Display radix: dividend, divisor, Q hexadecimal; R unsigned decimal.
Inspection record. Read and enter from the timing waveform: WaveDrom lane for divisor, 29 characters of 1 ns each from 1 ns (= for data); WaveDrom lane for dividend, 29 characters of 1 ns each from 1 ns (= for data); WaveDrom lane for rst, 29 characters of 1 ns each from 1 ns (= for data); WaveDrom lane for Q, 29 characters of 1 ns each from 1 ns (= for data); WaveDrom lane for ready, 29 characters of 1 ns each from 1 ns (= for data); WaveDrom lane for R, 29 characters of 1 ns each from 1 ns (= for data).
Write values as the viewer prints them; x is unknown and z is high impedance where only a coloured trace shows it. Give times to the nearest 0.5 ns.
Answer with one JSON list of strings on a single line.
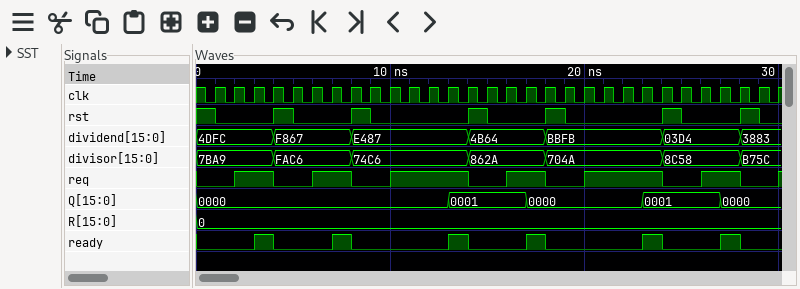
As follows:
["{name: 'divisor', wave: '=..=...=.....=...=.....=...=.', data: '7BA9 FAC6 74C6 862A 704A 8C58 B75C'}", "{name: 'dividend', wave: '=..=...=.....=...=.....=...=.', data: '4DFC F867 E487 4B64 BBFB 03D4 3883'}", "{name: 'rst', wave: '0..10..10....10..10....10..10'}", "{name: 'Q', wave: '=...........=...=.....=...=..', data: '0000 0001 0000 0001 0000'}", "{name: 'ready', wave: '0.10..10....10..10....10..10.'}", "{name: 'R', wave: '=............................', data: '0'}"]
